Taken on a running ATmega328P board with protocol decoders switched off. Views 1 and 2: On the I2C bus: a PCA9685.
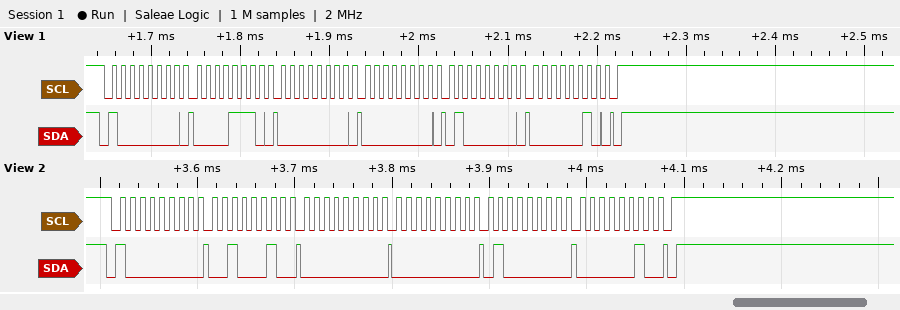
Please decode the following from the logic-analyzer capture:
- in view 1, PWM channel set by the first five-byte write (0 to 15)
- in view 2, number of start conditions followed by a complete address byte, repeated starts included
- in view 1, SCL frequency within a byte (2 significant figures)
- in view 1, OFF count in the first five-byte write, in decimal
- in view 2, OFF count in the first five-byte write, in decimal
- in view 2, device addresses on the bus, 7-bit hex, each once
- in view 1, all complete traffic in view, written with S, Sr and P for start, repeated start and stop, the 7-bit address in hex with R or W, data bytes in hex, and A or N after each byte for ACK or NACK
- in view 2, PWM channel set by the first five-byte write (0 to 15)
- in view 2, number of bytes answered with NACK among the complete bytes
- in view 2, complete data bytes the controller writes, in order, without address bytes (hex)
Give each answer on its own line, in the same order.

2
1
100 kHz
576
576
0x40
S 40W A 0E A 00 A 00 A 40 A 02 A P
7
0
22 00 00 40 02
